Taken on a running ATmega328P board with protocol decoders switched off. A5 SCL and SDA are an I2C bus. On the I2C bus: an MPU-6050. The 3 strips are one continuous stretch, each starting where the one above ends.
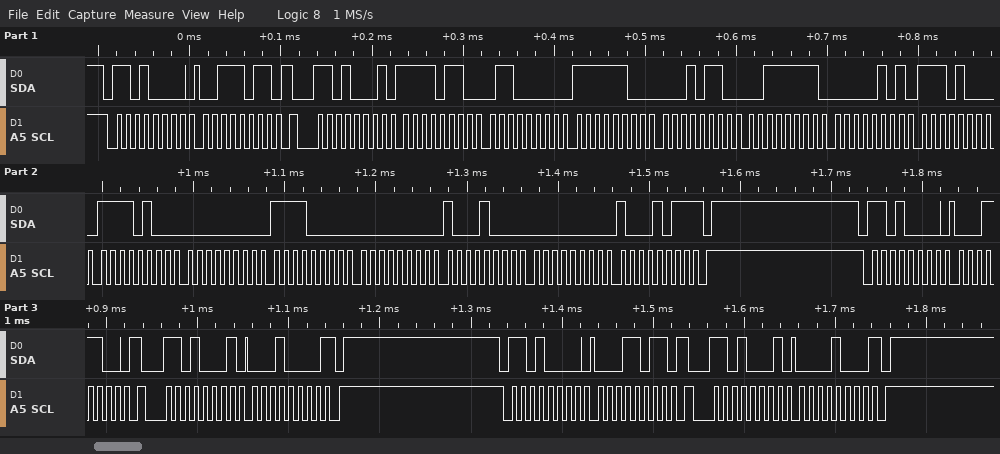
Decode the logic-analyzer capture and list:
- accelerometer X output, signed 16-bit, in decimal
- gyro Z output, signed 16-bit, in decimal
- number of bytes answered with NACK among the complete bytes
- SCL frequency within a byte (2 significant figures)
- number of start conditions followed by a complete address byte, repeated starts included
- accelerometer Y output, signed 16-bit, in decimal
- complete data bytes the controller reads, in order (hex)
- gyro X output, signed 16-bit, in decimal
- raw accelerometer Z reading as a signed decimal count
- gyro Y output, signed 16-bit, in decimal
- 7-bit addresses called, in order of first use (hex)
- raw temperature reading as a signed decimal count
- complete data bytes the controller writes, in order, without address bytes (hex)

-2464
139
3
100 kHz
6
-1002
F6 60 FC 16 3F 05 E8 F4 00 F0 00 88 00 8B 10 08
240
16133
136
0x68
-5900
3B 1C 1B
